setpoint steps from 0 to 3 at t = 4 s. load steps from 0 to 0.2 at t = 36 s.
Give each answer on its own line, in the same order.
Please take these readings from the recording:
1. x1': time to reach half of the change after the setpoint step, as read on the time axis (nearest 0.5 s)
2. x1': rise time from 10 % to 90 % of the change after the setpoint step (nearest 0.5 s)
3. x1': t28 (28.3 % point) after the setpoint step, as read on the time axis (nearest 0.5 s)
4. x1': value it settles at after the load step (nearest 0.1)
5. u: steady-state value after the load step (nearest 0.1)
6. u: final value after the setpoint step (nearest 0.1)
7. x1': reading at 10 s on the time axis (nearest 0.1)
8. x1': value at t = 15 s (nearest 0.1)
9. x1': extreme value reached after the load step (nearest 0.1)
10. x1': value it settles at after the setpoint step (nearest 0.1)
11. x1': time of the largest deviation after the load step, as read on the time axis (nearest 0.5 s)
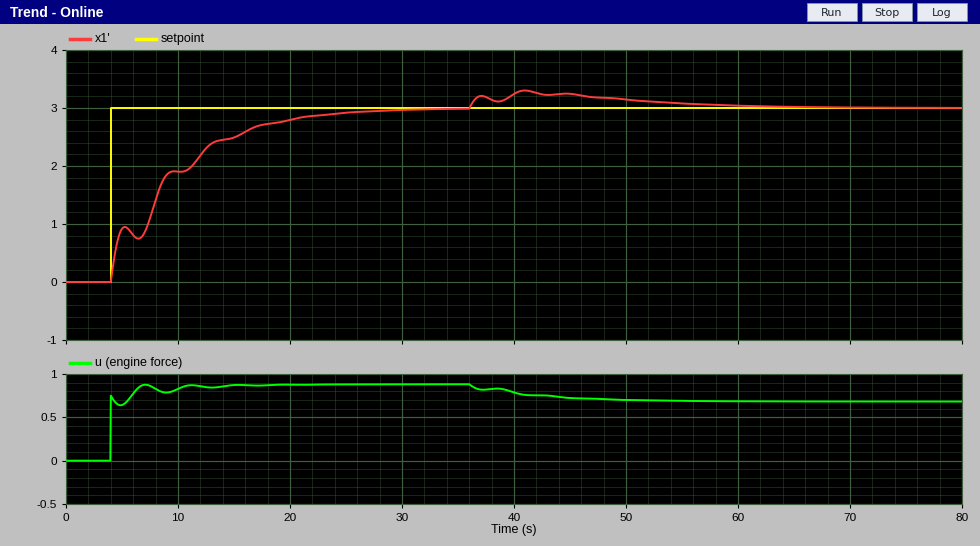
8.0 s
13.0 s
5.0 s
3.0
0.7
0.9
1.9
2.5
3.3
3.0
41.0 s
